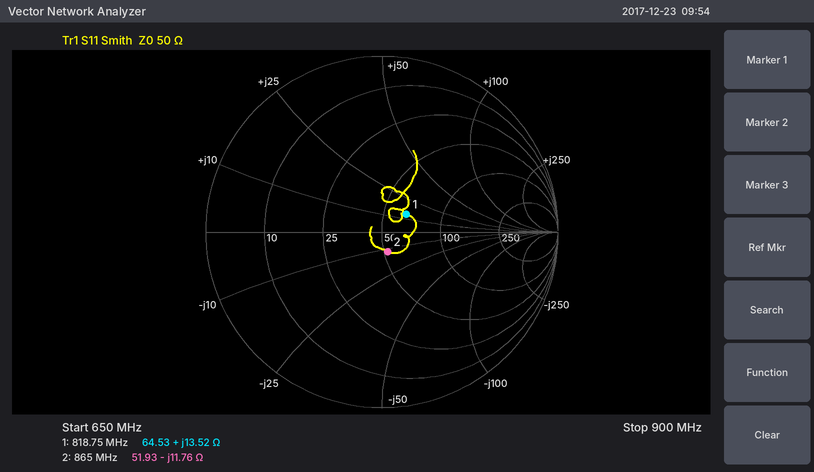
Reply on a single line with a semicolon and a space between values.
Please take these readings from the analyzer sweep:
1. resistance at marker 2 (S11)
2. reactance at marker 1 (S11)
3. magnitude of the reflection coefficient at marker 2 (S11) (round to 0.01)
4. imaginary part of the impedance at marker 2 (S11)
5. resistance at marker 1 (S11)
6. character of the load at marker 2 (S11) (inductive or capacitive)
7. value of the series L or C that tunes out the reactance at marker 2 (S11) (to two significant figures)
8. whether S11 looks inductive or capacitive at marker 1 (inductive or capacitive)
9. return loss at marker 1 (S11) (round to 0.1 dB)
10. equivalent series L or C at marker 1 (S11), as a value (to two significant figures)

51.93 Ω; +13.52 Ω; 0.12; -11.76 Ω; 64.53 Ω; capacitive; 2.2 nH; inductive; 15.3 dB; 2.6 nH
